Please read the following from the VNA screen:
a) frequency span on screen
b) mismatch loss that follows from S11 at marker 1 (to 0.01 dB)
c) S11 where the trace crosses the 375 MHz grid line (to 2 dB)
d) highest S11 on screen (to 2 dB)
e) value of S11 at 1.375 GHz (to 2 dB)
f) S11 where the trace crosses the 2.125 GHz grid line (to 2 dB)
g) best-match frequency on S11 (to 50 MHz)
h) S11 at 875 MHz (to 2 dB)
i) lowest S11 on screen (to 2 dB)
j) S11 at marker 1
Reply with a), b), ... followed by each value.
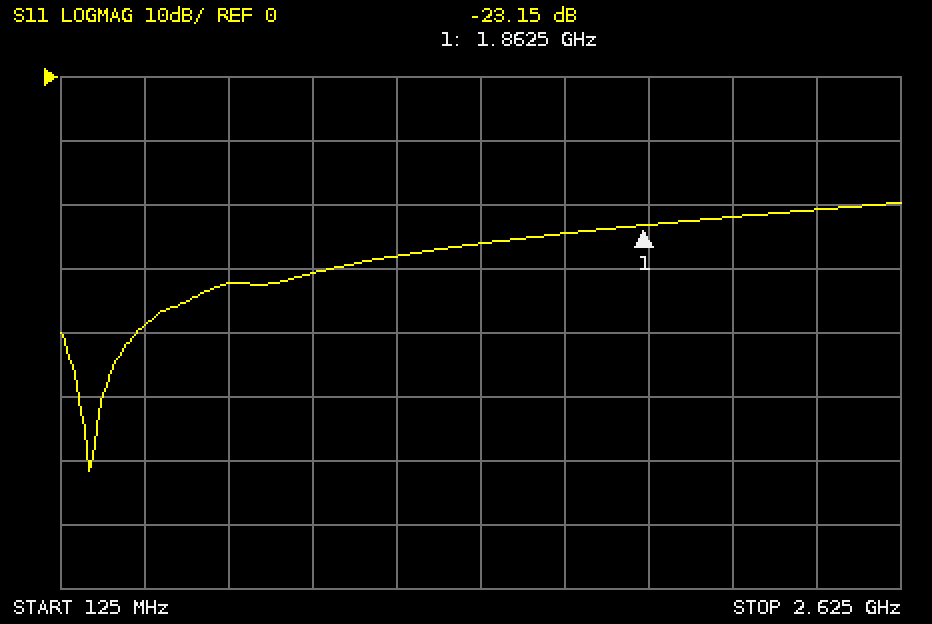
a) 2.5 GHz
b) 0.02 dB
c) -38 dB
d) -20 dB
e) -26 dB
f) -22 dB
g) 200 MHz
h) -30 dB
i) -62 dB
j) -23.15 dB
